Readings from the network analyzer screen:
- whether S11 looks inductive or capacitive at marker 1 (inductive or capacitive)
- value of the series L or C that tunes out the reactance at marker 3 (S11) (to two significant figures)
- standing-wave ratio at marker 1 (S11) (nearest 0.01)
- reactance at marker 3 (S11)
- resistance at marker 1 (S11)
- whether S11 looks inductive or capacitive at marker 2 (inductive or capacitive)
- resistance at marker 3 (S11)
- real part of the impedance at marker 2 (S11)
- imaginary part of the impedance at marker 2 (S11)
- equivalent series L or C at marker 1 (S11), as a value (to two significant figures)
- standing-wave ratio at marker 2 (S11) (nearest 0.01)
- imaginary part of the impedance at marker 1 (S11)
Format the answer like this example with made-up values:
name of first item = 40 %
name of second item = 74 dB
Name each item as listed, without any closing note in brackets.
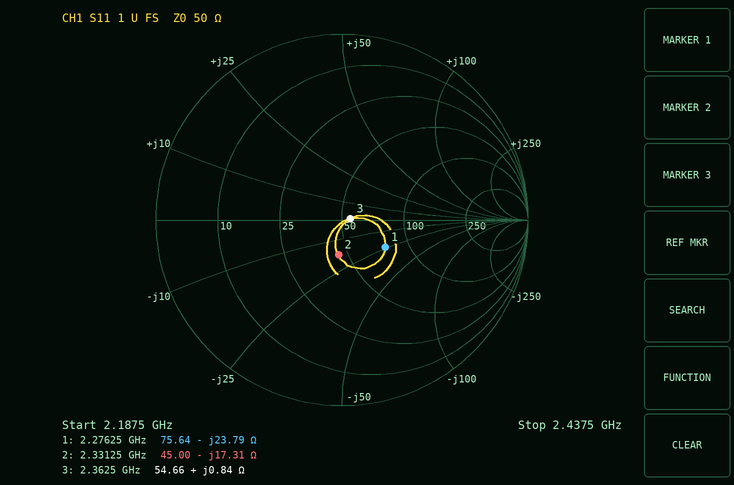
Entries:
whether S11 looks inductive or capacitive at marker 1 = capacitive
value of the series L or C that tunes out the reactance at marker 3 (S11) = 80 pF
standing-wave ratio at marker 1 (S11) = 1.75
reactance at marker 3 = +0.84 Ω
resistance at marker 1 = 75.64 Ω
whether S11 looks inductive or capacitive at marker 2 = capacitive
resistance at marker 3 = 54.66 Ω
real part of the impedance at marker 2 = 45.00 Ω
imaginary part of the impedance at marker 2 = -17.31 Ω
equivalent series L or C at marker 1 (S11), as a value = 2.9 pF
standing-wave ratio at marker 2 (S11) = 1.46
imaginary part of the impedance at marker 1 = -23.79 Ω
